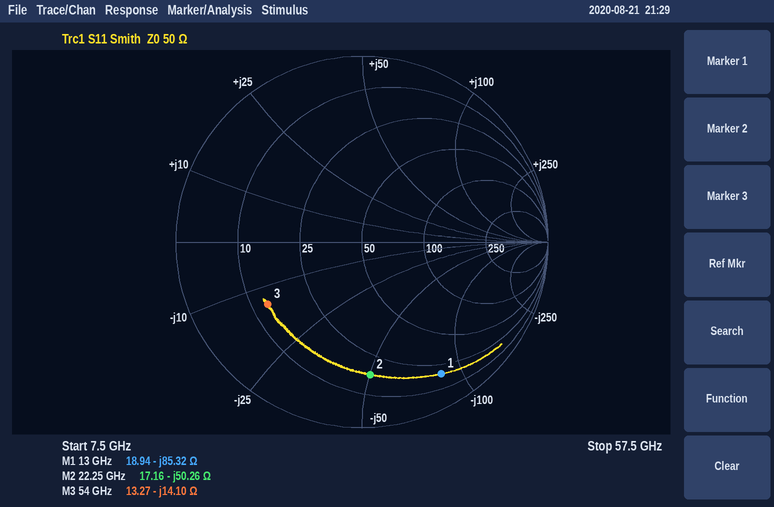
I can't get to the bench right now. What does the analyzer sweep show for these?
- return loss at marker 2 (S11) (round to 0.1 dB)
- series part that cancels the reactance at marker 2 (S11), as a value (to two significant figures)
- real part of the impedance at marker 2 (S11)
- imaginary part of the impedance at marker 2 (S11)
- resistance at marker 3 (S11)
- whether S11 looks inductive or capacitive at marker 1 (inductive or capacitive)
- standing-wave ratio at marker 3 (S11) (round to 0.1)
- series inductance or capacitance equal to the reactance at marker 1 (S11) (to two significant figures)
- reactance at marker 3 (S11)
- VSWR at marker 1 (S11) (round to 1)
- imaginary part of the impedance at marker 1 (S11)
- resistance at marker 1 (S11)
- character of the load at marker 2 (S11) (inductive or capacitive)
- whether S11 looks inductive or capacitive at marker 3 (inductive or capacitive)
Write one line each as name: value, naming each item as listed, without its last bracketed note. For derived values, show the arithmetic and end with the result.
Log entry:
return loss at marker 2 (S11): 2.9 dB
series part that cancels the reactance at marker 2 (S11), as a value: L = 50.26 Ω/(2π × 22.25 GHz) ≈ 360 pH
real part of the impedance at marker 2: 17.16 Ω
imaginary part of the impedance at marker 2: -50.26 Ω
resistance at marker 3: 13.27 Ω
whether S11 looks inductive or capacitive at marker 1: capacitive
standing-wave ratio at marker 3 (S11): 4.1
series inductance or capacitance equal to the reactance at marker 1 (S11): C = 1/(2π × 13 GHz × 85.32 Ω) ≈ 143 fF, so 140 fF to two significant figures
reactance at marker 3: -14.10 Ω
VSWR at marker 1 (S11): 11
imaginary part of the impedance at marker 1: -85.32 Ω
resistance at marker 1: 18.94 Ω
character of the load at marker 2 (S11): capacitive
whether S11 looks inductive or capacitive at marker 3: capacitive
